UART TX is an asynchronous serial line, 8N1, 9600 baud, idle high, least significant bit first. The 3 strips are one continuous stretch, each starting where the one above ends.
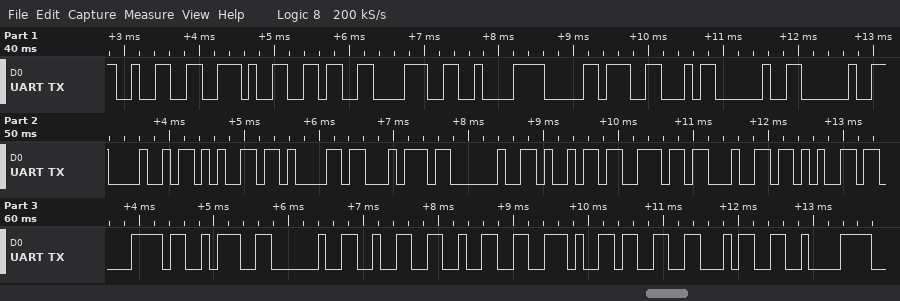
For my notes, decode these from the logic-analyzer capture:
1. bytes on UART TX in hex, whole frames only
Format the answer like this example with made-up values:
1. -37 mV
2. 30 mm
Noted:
1. 0x32 0x2E 0x36 0x38 0xC2 0xB0 0x46 0x20 0x20 0x48 0x65 0x61 0x74 0x20 0x69 0x6E 0x64 0x65 0x78 0x3A 0x20 0x32 0x32 0x2E 0x33 0x34 0xC2
